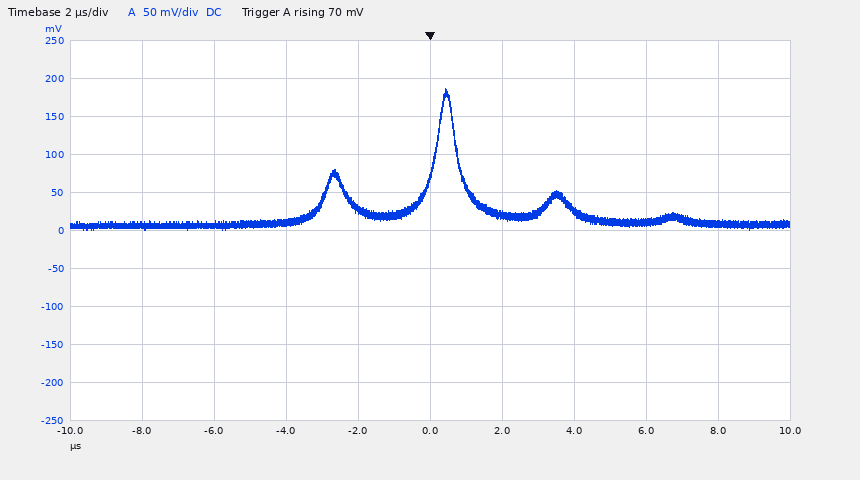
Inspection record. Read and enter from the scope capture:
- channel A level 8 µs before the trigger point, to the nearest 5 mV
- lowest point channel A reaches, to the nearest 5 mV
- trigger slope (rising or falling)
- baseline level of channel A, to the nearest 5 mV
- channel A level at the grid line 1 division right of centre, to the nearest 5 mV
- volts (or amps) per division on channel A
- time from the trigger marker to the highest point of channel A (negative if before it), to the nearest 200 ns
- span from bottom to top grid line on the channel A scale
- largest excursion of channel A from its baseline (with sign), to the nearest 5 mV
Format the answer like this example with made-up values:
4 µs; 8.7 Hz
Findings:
5 mV; 0 mV; rising; 10 mV; 20 mV; 50 mV; +400 ns; 500 mV; +180 mV
